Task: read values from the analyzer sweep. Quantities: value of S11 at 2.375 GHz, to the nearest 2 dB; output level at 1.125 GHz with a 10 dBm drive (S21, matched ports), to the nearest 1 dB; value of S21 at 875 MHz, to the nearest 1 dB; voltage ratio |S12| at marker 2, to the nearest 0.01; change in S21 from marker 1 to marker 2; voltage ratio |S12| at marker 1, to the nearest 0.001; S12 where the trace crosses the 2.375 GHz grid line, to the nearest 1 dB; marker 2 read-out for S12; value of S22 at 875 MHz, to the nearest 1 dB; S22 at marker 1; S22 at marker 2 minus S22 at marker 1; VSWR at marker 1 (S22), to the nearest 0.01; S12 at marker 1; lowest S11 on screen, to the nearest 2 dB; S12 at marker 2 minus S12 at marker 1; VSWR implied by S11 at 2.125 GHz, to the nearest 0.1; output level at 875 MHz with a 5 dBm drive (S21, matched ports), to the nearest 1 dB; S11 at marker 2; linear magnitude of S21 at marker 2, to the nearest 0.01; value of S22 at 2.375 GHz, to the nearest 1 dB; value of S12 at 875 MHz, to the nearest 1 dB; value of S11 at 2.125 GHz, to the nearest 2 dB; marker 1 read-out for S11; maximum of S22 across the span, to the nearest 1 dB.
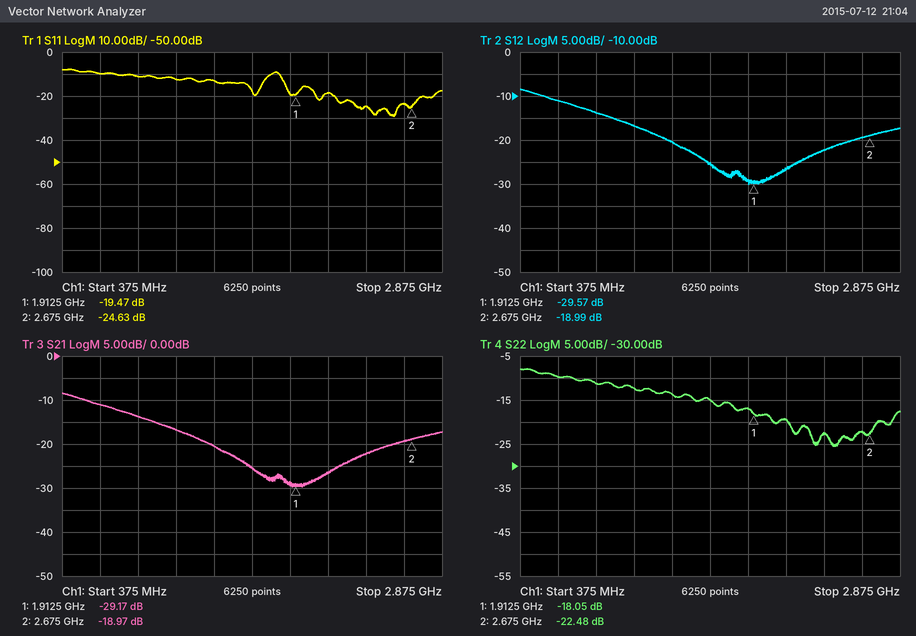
-24 dB
-7 dBm
-14 dB
0.11
10.20 dB
0.033
-22 dB
-18.99 dB
-11 dB
-18.05 dB
-4.43 dB
1.29
-29.57 dB
-30 dB
10.58 dB
1.3
-9 dBm
-24.63 dB
0.11
-23 dB
-14 dB
-18 dB
-19.47 dB
-8 dB
